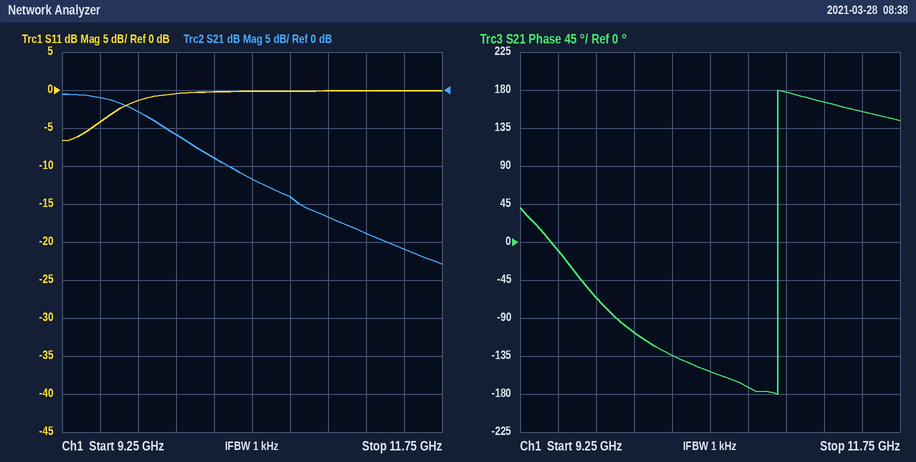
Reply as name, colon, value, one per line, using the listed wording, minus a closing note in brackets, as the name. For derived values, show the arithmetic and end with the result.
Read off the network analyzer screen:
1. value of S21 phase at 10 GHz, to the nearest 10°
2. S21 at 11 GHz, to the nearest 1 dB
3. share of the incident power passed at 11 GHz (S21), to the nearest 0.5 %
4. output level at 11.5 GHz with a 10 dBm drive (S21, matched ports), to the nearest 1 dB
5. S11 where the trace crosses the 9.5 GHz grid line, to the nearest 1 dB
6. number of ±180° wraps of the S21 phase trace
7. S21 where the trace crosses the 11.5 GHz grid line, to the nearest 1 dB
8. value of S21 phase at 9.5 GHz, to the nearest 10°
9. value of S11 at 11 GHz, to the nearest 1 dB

value of S21 phase at 10 GHz, to the nearest 10°: -110°
S21 at 11 GHz, to the nearest 1 dB: -17 dB
share of the incident power passed at 11 GHz (S21), to the nearest 0.5 %: 10^(-17/10) ≈ 2.0 %
output level at 11.5 GHz with a 10 dBm drive (S21, matched ports), to the nearest 1 dB: 10 dBm + (-21 dB) = -11 dBm
S11 where the trace crosses the 9.5 GHz grid line, to the nearest 1 dB: -4 dB
number of ±180° wraps of the S21 phase trace: 1
S21 where the trace crosses the 11.5 GHz grid line, to the nearest 1 dB: -21 dB
value of S21 phase at 9.5 GHz, to the nearest 10°: -10°
value of S11 at 11 GHz, to the nearest 1 dB: 0 dB
